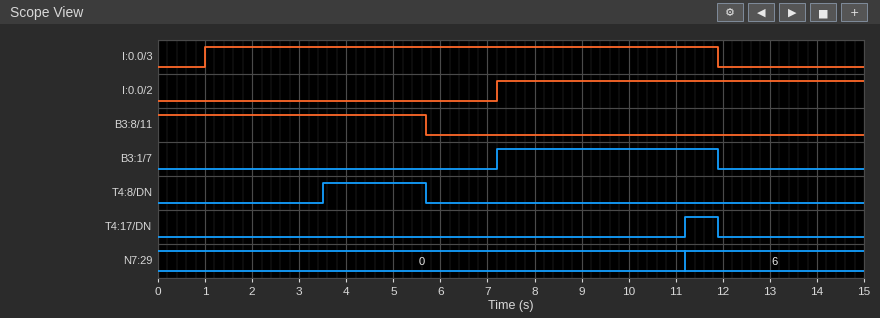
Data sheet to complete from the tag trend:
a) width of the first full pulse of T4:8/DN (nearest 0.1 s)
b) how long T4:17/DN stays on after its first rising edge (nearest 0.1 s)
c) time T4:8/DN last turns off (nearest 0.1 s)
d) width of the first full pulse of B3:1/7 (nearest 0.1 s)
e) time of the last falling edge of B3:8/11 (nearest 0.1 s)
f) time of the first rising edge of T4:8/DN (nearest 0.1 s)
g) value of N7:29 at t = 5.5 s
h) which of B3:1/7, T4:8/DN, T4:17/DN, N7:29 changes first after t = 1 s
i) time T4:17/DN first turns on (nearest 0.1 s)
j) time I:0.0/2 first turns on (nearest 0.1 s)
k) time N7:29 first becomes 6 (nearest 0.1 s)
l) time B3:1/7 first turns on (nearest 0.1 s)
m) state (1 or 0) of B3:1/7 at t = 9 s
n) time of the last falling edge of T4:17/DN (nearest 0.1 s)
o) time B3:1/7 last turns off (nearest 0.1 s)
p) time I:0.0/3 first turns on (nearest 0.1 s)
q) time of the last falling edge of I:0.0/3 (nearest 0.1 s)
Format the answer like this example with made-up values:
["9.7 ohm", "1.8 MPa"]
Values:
["2.2 s", "0.7 s", "5.7 s", "4.7 s", "5.7 s", "3.5 s", "0", "T4:8/DN", "11.2 s", "7.2 s", "11.2 s", "7.2 s", "1", "11.9 s", "11.9 s", "1.0 s", "11.9 s"]
